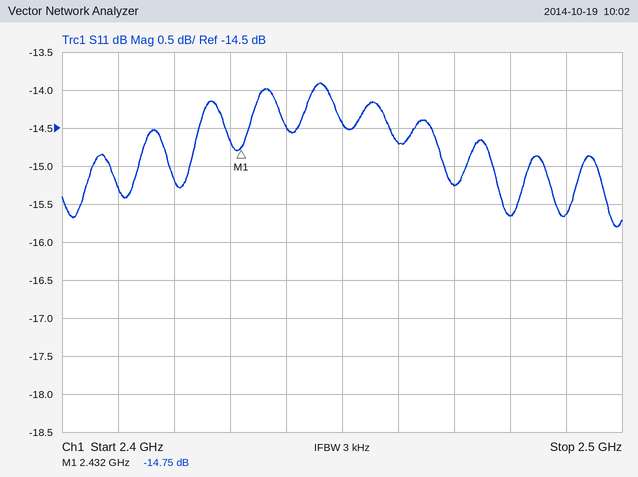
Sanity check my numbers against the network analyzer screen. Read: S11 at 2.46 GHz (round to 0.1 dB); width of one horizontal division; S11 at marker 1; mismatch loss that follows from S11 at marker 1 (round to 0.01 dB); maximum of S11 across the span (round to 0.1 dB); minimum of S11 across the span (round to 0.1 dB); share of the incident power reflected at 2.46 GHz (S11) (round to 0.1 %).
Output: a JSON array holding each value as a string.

["-14.7 dB", "10 MHz", "-14.75 dB", "0.15 dB", "-13.9 dB", "-15.8 dB", "3.4 %"]
